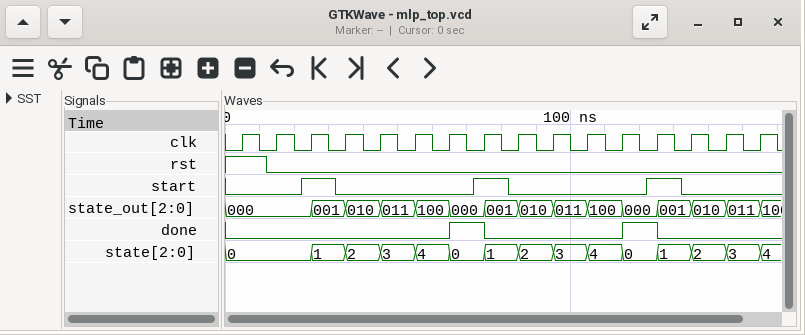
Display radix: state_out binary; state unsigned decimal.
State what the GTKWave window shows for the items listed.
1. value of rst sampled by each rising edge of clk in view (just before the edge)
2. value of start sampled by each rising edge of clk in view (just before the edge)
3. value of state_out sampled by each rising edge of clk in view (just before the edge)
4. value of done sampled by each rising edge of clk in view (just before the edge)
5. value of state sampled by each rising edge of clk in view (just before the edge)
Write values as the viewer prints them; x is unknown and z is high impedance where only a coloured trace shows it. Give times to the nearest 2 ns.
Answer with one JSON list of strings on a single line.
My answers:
["1 0 0 0 0 0 0 0 0 0 0 0 0 0 0 0", "0 0 1 0 0 0 0 1 0 0 0 0 1 0 0 0", "000, 000, 000, 001, 010, 011, 100, 000, 001, 010, 011, 100, 000, 001, 010, 011", "0 0 0 0 0 0 0 1 0 0 0 0 1 0 0 0", "0, 0, 0, 1, 2, 3, 4, 0, 1, 2, 3, 4, 0, 1, 2, 3"]
